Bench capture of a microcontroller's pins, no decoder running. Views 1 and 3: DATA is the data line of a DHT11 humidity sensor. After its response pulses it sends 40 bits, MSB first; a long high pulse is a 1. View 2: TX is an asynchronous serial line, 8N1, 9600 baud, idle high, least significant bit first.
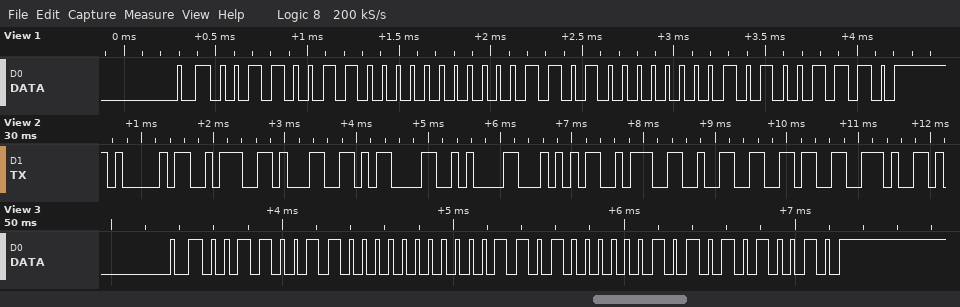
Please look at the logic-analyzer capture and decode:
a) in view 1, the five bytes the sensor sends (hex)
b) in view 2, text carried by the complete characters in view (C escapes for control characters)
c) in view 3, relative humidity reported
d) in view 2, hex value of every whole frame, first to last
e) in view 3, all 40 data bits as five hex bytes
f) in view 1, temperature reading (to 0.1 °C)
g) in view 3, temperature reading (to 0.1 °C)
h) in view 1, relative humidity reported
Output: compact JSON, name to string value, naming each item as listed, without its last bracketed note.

{"in view 1, the five bytes the sensor sends": "33 00 1A 01 4E", "in view 2, text carried by the complete characters in view": "\"A:1\\r\\nT:26.\"", "in view 3, relative humidity reported": "51 %", "in view 2, hex value of every whole frame, first to last": "41 3A 31 0D 0A 54 3A 32 36 2E", "in view 3, all 40 data bits as five hex bytes": "33 00 1A 05 52", "in view 1, temperature reading": "26.1 °C", "in view 3, temperature reading": "26.5 °C", "in view 1, relative humidity reported": "51 %"}
